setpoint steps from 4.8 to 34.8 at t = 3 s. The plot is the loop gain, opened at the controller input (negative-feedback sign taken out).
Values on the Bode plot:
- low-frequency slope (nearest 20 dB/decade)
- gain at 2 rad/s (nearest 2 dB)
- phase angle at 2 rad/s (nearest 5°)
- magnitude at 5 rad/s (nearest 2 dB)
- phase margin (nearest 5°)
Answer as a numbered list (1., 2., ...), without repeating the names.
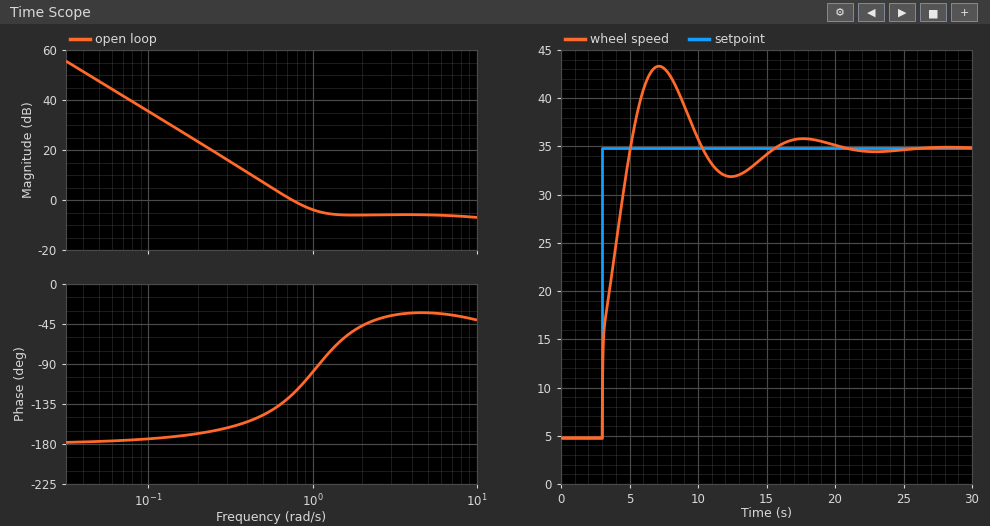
1. -40 dB/decade
2. -6 dB
3. -45°
4. -6 dB
5. 55°
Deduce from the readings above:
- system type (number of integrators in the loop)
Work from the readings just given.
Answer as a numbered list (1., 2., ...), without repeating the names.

1. 2
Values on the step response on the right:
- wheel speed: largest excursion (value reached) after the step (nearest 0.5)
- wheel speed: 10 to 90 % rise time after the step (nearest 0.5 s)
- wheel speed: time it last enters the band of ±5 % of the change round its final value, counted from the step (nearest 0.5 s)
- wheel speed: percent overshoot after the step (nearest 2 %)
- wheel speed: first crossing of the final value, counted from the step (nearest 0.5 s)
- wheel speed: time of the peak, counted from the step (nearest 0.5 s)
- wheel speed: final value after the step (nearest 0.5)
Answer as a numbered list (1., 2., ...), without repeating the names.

1. 43.5
2. 1.5 s
3. 11.5 s
4. 28 %
5. 2.0 s
6. 4.0 s
7. 35.0
